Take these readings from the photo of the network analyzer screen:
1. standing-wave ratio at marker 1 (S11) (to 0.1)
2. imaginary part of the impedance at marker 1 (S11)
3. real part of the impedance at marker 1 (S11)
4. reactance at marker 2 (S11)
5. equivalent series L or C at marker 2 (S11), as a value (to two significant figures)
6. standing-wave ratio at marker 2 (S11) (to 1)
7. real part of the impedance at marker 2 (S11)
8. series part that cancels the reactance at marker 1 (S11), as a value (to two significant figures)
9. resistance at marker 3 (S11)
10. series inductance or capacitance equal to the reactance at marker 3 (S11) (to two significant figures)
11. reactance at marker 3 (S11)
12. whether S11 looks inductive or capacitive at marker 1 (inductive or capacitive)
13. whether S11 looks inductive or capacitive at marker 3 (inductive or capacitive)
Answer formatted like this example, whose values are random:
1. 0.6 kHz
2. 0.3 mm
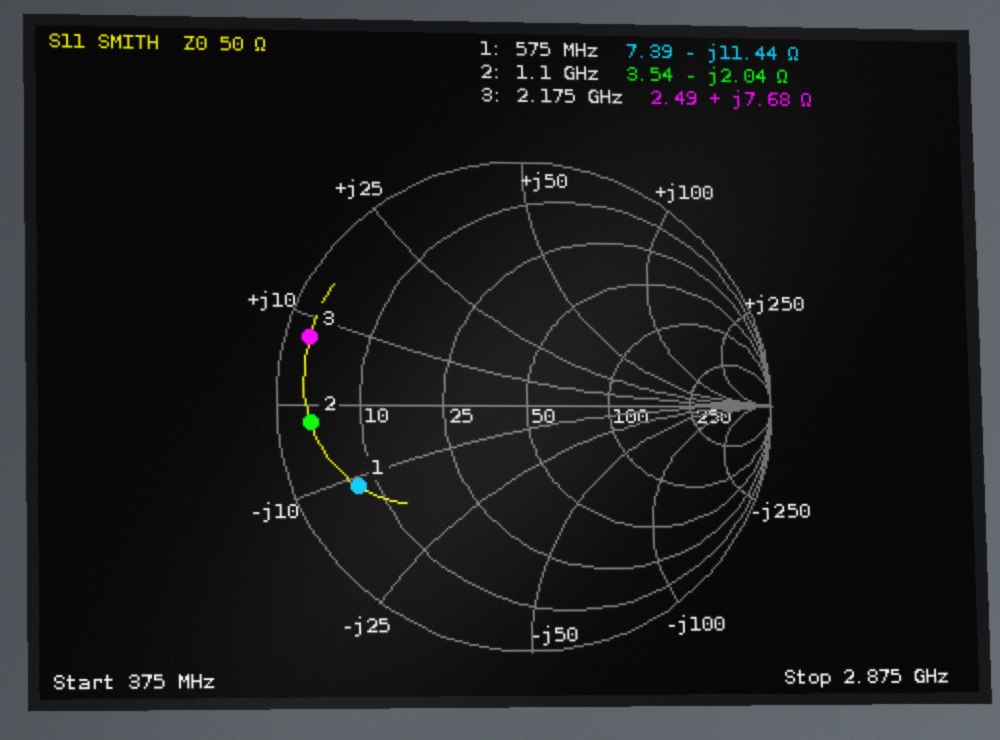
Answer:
1. 7.1
2. -11.44 Ω
3. 7.39 Ω
4. -2.04 Ω
5. 71 pF
6. 14
7. 3.54 Ω
8. 3.2 nH
9. 2.49 Ω
10. 560 pH
11. +7.68 Ω
12. capacitive
13. inductive
